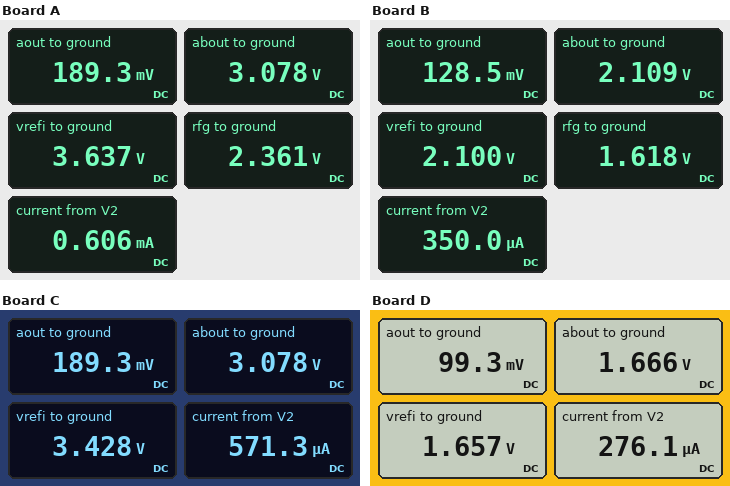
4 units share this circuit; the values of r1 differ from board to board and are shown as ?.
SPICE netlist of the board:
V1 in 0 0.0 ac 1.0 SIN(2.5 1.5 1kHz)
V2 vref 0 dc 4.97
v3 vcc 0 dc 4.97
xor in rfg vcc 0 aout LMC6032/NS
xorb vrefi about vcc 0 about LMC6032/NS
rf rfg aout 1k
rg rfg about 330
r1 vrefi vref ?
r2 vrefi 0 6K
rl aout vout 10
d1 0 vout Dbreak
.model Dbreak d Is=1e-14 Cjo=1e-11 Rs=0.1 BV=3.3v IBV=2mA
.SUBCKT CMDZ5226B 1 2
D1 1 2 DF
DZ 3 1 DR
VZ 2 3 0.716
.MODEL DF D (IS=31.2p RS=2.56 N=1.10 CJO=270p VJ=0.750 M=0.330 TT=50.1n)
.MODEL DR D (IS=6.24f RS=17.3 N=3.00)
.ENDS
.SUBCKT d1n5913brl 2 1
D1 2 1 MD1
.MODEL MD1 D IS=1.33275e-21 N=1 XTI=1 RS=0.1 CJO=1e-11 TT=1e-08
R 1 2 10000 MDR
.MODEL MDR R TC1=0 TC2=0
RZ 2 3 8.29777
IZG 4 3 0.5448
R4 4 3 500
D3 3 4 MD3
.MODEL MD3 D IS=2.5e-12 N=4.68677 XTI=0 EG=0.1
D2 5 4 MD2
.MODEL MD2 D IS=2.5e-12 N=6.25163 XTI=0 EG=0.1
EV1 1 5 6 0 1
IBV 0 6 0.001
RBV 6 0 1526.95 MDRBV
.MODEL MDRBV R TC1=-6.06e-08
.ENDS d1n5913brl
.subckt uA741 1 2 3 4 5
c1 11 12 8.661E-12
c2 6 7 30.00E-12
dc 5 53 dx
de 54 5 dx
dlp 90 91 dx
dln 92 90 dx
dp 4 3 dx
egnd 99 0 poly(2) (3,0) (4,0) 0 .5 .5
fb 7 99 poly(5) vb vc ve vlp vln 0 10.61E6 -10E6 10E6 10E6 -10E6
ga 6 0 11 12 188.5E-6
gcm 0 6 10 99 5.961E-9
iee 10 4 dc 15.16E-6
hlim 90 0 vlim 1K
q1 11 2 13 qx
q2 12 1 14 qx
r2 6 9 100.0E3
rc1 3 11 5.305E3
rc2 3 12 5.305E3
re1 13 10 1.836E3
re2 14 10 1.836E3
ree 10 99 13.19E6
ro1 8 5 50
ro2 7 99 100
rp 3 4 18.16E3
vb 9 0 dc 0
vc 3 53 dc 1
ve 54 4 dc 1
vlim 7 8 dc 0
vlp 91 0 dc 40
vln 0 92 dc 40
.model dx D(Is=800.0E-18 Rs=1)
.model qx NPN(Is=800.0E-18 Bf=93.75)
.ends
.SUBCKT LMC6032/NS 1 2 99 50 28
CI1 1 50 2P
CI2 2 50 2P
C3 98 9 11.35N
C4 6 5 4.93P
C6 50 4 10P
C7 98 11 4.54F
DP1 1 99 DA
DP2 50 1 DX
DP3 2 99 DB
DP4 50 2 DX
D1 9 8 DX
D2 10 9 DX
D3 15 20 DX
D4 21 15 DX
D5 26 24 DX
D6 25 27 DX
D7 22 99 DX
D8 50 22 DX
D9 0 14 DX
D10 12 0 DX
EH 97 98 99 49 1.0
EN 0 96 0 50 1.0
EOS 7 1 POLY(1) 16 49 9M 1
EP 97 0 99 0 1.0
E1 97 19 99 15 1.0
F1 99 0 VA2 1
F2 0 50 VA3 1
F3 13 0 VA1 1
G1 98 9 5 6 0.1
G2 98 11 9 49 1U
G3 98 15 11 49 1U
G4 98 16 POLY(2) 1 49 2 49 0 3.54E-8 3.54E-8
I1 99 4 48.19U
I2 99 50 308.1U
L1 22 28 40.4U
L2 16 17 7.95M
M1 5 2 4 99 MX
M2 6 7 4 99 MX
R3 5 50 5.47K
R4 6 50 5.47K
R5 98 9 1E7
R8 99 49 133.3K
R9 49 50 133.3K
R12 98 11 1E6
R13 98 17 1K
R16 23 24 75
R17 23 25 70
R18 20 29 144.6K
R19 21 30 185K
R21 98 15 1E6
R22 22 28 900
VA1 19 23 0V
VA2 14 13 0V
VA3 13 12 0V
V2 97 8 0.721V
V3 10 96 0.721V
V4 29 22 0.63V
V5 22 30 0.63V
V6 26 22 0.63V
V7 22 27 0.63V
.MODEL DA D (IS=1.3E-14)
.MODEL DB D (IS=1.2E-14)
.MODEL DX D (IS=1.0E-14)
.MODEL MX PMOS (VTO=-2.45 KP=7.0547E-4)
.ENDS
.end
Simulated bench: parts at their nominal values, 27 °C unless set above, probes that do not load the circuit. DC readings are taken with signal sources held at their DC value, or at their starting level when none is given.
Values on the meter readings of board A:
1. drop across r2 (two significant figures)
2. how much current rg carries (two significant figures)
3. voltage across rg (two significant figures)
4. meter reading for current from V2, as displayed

3.6 V
2.2 mA
720 mV
0.606 mA
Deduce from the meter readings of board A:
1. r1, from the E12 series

2.2 kΩ
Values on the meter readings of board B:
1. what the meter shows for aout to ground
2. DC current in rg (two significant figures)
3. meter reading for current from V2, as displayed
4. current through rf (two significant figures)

128.5 mV
1.5 mA
350.0 µA
1.5 mA
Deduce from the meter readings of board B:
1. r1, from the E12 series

8.2 kΩ
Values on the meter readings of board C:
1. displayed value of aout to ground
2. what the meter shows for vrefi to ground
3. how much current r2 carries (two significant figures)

189.3 mV
3.428 V
570 µA
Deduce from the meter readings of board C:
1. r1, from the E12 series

2.7 kΩ
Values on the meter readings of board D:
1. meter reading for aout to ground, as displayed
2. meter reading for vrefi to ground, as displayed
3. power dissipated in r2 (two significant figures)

99.3 mV
1.657 V
460 µW
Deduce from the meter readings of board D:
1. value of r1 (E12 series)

12 kΩ
